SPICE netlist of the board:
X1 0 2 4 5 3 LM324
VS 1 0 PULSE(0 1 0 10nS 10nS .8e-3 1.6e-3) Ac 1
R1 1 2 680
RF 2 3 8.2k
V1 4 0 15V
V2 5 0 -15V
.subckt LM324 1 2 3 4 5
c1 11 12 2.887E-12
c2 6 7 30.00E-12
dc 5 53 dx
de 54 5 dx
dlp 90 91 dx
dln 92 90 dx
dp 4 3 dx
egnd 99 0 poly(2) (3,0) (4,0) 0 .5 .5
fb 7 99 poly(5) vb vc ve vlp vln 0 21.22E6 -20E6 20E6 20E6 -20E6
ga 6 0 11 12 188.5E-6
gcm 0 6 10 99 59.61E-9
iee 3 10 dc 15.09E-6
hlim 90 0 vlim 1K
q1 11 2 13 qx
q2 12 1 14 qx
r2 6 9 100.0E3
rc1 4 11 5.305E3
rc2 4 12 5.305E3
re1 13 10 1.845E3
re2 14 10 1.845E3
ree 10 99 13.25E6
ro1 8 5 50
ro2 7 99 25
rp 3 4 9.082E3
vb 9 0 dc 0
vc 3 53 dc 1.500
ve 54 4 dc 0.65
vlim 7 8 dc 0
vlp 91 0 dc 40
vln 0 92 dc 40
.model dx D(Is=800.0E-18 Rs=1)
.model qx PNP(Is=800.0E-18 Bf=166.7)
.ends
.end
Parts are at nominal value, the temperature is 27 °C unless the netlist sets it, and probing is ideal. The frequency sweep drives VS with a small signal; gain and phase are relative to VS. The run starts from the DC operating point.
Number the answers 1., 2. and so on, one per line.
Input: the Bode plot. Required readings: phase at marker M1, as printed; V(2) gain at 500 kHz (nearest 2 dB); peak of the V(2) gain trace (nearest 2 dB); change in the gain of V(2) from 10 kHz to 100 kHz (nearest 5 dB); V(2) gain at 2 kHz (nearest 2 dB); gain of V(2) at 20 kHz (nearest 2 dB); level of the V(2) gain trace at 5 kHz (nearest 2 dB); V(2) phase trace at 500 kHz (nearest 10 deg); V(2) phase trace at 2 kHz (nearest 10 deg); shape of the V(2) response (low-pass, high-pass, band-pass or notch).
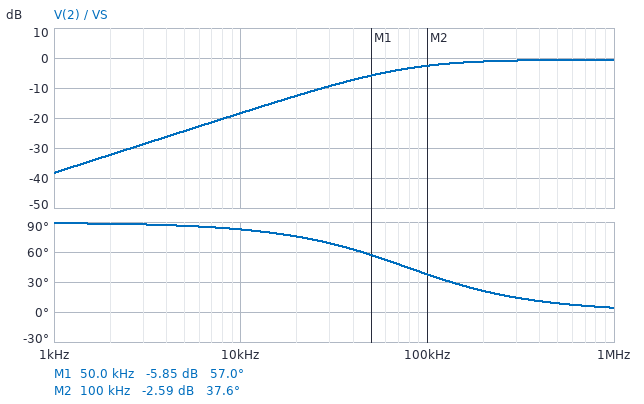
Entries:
1. 57.0 deg
2. 0 dB
3. 0 dB
4. 15 dB
5. -32 dB
6. -12 dB
7. -24 dB
8. 10 deg
9. 90 deg
10. high-pass
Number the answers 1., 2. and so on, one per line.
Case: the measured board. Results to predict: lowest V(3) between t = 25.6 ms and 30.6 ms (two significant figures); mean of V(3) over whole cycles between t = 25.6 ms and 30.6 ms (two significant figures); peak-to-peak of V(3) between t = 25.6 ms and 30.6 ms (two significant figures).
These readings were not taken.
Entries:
1. -12 V
2. -6.0 V
3. 12 V
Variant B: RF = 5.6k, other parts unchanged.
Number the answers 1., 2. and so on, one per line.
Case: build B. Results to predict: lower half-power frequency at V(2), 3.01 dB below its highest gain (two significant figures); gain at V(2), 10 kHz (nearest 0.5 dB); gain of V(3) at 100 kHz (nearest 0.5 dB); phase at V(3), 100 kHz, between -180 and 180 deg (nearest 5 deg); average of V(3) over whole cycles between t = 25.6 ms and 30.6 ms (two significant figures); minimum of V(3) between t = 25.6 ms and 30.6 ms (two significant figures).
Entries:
1. 110 kHz
2. -21.5 dB
3. 15.5 dB
4. 135 deg
5. -4.1 V
6. -8.2 V
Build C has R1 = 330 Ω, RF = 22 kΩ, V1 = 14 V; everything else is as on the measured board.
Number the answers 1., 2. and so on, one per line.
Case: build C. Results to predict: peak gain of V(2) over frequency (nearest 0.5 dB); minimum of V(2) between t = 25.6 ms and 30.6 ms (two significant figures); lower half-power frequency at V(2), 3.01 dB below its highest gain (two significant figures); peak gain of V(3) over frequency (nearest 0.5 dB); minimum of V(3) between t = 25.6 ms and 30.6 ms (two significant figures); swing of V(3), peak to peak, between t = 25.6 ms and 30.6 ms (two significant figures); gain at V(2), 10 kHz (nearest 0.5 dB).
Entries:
1. 0 dB
2. -220 mV
3. 15 kHz
4. 36.5 dB
5. -15 V
6. 15 V
7. -5.0 dB
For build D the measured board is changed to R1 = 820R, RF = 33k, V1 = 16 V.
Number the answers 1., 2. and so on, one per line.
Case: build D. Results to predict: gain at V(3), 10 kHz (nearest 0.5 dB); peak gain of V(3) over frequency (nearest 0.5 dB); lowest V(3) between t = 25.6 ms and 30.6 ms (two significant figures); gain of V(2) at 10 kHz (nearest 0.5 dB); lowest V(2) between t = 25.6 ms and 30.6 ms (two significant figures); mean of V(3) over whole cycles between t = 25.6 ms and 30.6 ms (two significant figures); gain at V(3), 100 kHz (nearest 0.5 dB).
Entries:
1. 31.5 dB
2. 32.0 dB
3. -15 V
4. -8.5 dB
5. -360 mV
6. -7.5 V
7. 19.5 dB
